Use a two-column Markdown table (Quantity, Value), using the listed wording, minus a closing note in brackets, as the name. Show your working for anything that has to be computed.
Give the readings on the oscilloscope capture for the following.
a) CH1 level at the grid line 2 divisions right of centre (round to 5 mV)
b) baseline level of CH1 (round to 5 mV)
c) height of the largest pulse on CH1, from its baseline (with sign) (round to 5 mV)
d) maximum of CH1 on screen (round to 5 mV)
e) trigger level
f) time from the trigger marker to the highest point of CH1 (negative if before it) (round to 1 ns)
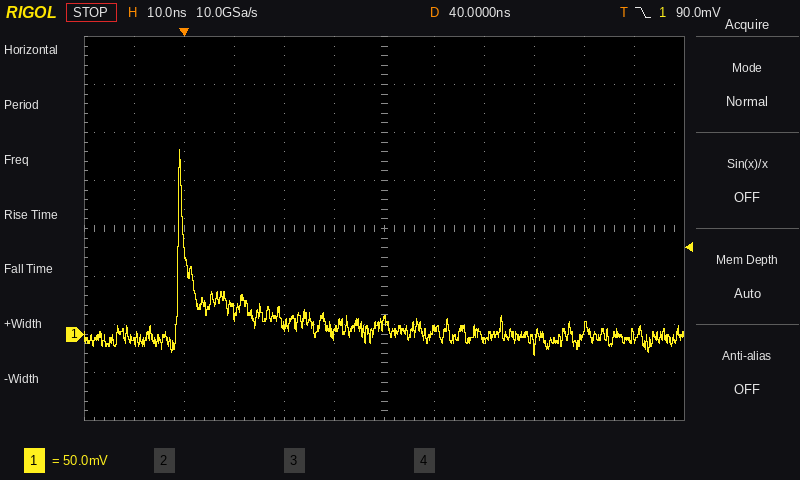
| Quantity | Value |
|---|---|
| CH1 level at the grid line 2 divisions right of centre | -5 mV |
| baseline level of CH1 | 0 mV |
| height of the largest pulse on CH1, from its baseline (with sign) | 190 mV − (0 mV) = +190 mV |
| maximum of CH1 on screen | 190 mV |
| trigger level | 90.0 mV |
| time from the trigger marker to the highest point of CH1 (negative if before it) | -1 ns |
